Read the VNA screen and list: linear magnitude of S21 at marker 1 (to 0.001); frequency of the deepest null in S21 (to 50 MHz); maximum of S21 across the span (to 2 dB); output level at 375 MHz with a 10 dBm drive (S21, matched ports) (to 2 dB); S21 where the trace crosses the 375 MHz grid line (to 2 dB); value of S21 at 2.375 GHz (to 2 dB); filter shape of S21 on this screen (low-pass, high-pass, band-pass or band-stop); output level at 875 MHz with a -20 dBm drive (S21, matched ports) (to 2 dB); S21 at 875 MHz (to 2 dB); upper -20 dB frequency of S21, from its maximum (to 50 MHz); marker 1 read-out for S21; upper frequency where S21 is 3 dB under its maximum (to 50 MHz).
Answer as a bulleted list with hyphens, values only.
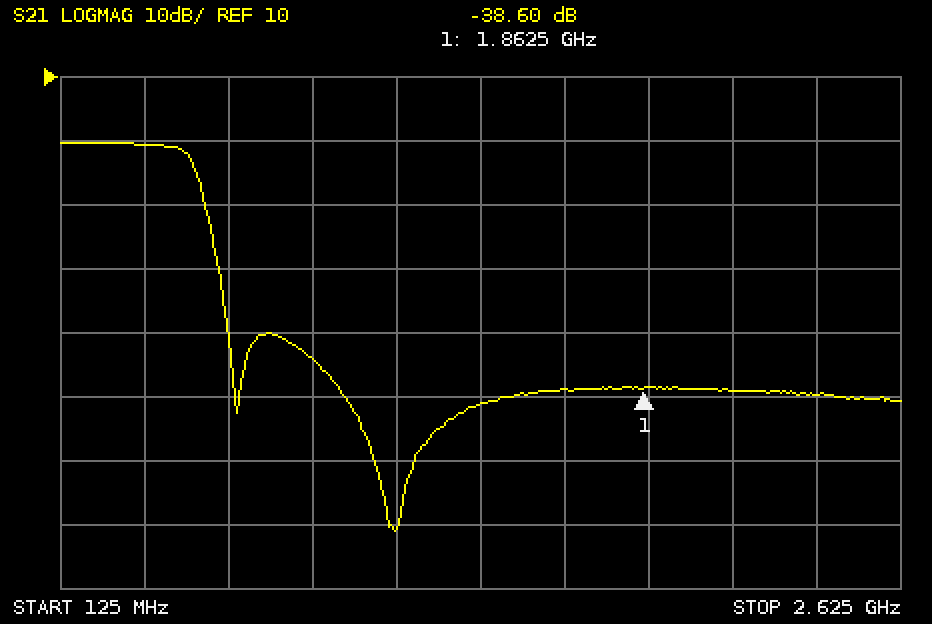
- 0.012
- 1.10 GHz
- 0 dB
- 10 dBm
- 0 dB
- -40 dB
- low-pass
- -54 dBm
- -34 dB
- 600 MHz
- -38.60 dB
- 500 MHz
